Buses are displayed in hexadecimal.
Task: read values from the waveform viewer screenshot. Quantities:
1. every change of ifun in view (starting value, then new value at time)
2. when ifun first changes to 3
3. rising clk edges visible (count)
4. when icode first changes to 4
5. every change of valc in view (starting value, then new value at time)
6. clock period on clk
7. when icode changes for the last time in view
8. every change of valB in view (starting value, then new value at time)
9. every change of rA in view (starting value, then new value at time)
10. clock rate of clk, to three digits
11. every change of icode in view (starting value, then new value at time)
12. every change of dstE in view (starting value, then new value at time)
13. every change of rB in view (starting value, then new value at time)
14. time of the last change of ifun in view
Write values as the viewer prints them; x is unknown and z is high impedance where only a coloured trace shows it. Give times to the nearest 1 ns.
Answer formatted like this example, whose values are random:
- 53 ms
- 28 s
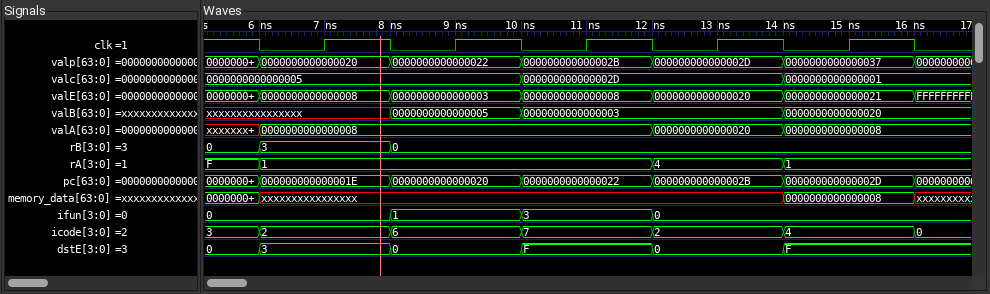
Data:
- 0, 1 at 8 ns, 3 at 10 ns, 0 at 12 ns
- 10 ns
- 5
- 14 ns
- 0000000000000005, 000000000000002D at 10 ns, 0000000000000001 at 14 ns
- 2 ns
- 16 ns
- xxxxxxxxxxxxxxxx, 0000000000000005 at 8 ns, 0000000000000003 at 10 ns, 0000000000000020 at 14 ns
- F, 1 at 6 ns, 4 at 12 ns, 1 at 14 ns
- 500 MHz
- 3, 2 at 6 ns, 6 at 8 ns, 7 at 10 ns, 2 at 12 ns, 4 at 14 ns, 0 at 16 ns
- 0, 3 at 6 ns, 0 at 8 ns, F at 10 ns, 0 at 12 ns, F at 14 ns
- 0, 3 at 6 ns, 0 at 8 ns
- 12 ns
